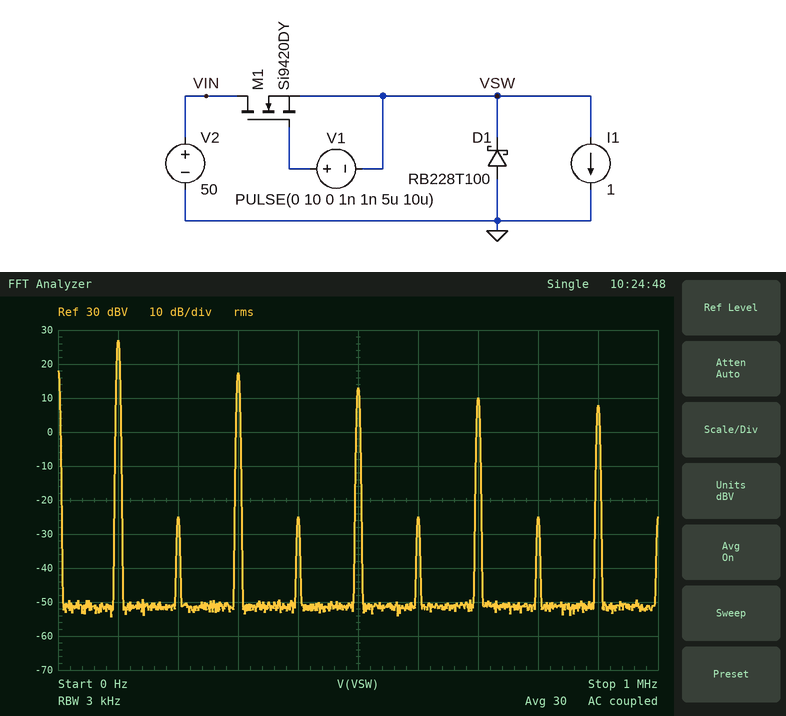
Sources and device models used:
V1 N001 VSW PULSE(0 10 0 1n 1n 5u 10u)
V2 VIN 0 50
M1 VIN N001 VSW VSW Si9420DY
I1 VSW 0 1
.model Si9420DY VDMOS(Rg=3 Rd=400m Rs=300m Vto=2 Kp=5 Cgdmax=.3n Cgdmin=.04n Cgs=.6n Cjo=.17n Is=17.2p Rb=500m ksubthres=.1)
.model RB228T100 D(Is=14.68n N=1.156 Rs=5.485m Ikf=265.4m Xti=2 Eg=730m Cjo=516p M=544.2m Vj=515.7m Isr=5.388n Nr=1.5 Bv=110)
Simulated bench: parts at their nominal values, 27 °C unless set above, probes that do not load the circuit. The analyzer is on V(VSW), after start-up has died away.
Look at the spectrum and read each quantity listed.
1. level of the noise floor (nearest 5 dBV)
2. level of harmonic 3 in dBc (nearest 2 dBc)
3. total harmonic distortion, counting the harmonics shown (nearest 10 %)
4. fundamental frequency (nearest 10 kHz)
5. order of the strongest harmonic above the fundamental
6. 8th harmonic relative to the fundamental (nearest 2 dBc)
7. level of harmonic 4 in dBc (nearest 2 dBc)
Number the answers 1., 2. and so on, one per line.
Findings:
1. -50 dBV
2. -10 dBc
3. 40 %
4. 100 kHz
5. 3
6. -52 dBc
7. -52 dBc
